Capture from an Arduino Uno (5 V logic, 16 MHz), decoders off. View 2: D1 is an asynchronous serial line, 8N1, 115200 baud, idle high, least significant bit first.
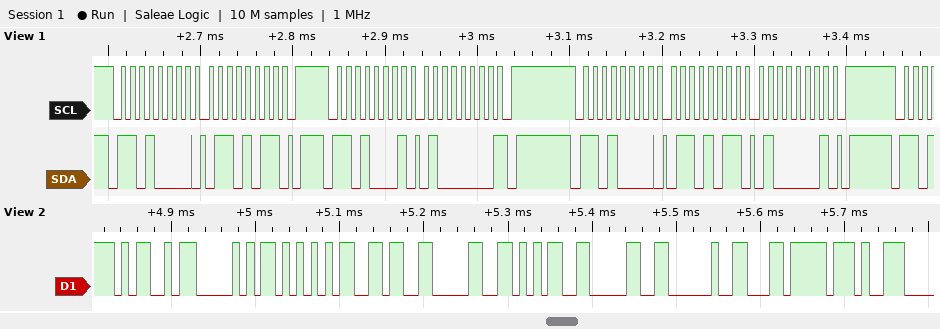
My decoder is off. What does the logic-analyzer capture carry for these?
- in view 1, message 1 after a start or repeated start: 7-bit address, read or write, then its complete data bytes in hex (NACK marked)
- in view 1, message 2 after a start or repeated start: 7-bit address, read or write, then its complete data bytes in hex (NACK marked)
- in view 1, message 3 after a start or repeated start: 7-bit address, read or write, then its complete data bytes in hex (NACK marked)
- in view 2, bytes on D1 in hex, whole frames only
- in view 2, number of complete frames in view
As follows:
0x68 write: 6B
0x68 read: 40 NACK
0x68 write: 6B 41
4D 50 55 36 30 35 30 20 EC 97
10
